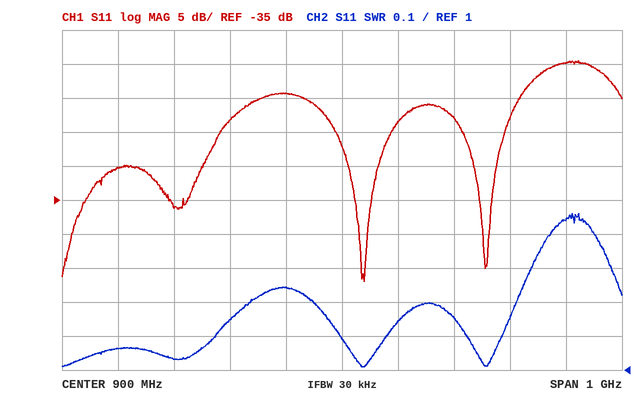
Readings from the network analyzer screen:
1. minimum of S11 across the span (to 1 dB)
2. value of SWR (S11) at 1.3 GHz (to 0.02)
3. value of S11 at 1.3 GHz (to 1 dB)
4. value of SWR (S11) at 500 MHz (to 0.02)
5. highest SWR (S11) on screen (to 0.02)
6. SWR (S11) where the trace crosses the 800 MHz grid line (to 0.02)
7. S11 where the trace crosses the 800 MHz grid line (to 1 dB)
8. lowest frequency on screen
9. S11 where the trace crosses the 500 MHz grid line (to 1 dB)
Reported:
-47 dB
1.44
-15 dB
1.06
1.46
1.24
-19 dB
400 MHz
-30 dB
